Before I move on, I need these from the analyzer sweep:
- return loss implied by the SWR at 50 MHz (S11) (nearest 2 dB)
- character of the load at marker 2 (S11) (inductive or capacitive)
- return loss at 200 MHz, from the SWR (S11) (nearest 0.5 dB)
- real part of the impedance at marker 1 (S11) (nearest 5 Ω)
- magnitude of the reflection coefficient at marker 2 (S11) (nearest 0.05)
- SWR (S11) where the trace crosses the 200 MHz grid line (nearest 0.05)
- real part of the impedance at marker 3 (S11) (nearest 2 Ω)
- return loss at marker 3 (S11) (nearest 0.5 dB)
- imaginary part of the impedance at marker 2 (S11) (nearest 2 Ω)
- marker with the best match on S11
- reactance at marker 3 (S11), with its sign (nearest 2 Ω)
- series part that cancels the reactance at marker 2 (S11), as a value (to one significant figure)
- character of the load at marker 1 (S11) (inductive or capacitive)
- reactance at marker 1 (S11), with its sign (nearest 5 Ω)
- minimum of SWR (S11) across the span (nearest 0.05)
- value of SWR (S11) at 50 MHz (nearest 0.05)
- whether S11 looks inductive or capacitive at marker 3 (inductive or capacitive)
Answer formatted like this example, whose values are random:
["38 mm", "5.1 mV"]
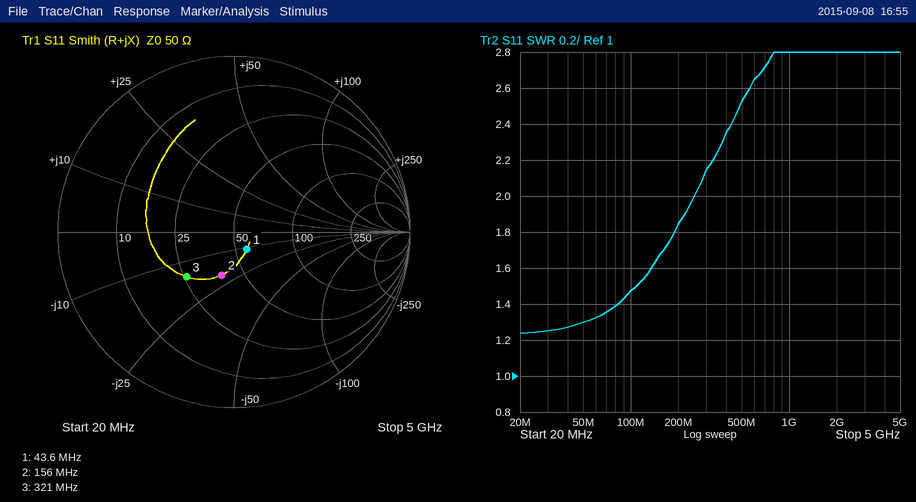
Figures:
["18 dB", "capacitive", "10.5 dB", "55 Ω", "0.25", "1.85", "26 Ω", "8.5 dB", "-20 Ω", "marker 1", "-16 Ω", "20 nH", "capacitive", "-10 Ω", "1.25", "1.30", "capacitive"]
